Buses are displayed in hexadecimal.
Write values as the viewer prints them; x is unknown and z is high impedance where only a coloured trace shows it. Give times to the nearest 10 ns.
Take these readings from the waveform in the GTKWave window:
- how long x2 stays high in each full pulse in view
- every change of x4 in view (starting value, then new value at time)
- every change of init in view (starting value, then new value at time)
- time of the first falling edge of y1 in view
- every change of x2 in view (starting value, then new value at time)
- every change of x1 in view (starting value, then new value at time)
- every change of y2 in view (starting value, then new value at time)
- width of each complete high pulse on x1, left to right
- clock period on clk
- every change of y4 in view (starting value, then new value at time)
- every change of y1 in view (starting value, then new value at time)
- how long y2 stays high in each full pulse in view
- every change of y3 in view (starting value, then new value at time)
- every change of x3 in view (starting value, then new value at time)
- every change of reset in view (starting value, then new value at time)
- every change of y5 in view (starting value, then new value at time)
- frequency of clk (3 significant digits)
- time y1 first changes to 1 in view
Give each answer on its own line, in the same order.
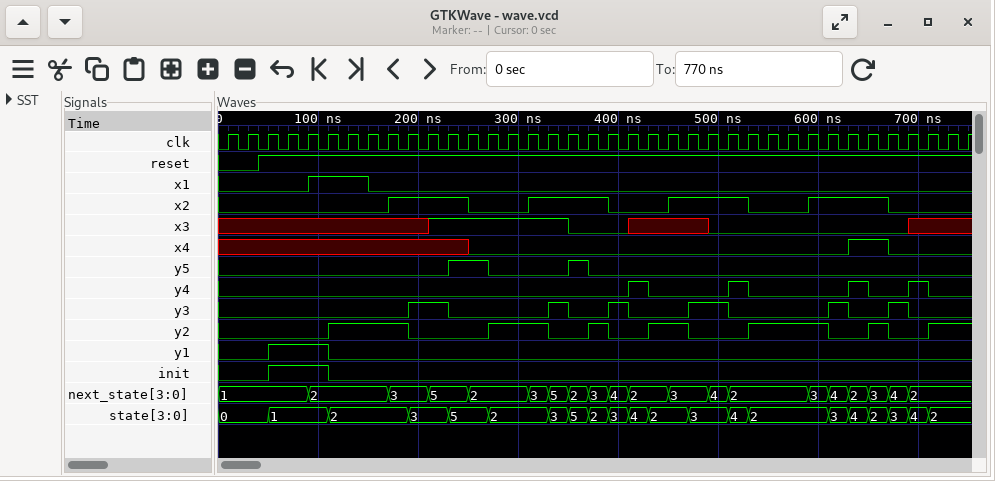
80 ns, 80 ns, 80 ns, 80 ns
x, 0 at 250 ns, 1 at 630 ns, 0 at 670 ns
0, 1 at 50 ns, 0 at 110 ns
110 ns
0, 1 at 170 ns, 0 at 250 ns, 1 at 310 ns, 0 at 390 ns, 1 at 450 ns, 0 at 530 ns, 1 at 590 ns, 0 at 670 ns
0, 1 at 90 ns, 0 at 150 ns
0, 1 at 110 ns, 0 at 190 ns, 1 at 270 ns, 0 at 330 ns, 1 at 370 ns, 0 at 390 ns, 1 at 430 ns, 0 at 470 ns, 1 at 530 ns, 0 at 610 ns, 1 at 650 ns, 0 at 670 ns, 1 at 710 ns
60 ns
20 ns
0, 1 at 410 ns, 0 at 430 ns, 1 at 510 ns, 0 at 530 ns, 1 at 630 ns, 0 at 650 ns, 1 at 690 ns, 0 at 710 ns
0, 1 at 50 ns, 0 at 110 ns
80 ns, 60 ns, 20 ns, 40 ns, 80 ns, 20 ns
0, 1 at 190 ns, 0 at 230 ns, 1 at 330 ns, 0 at 350 ns, 1 at 390 ns, 0 at 410 ns, 1 at 470 ns, 0 at 510 ns, 1 at 610 ns, 0 at 630 ns, 1 at 670 ns, 0 at 690 ns
x, 1 at 210 ns, 0 at 350 ns, x at 410 ns, 0 at 490 ns, x at 690 ns
0, 1 at 40 ns
0, 1 at 230 ns, 0 at 270 ns, 1 at 350 ns, 0 at 370 ns
50.0 MHz
50 ns
